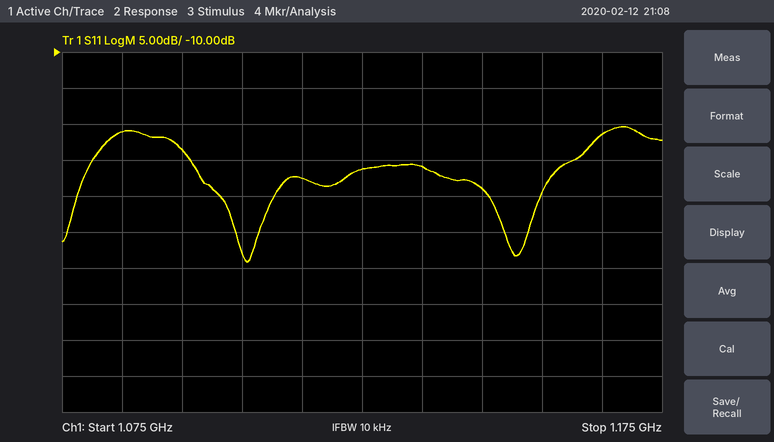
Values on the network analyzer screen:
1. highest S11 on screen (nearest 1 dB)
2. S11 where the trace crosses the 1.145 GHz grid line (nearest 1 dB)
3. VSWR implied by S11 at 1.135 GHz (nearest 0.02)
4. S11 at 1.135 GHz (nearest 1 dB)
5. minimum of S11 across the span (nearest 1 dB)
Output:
-20 dB
-29 dB
1.10
-26 dB
-39 dB
